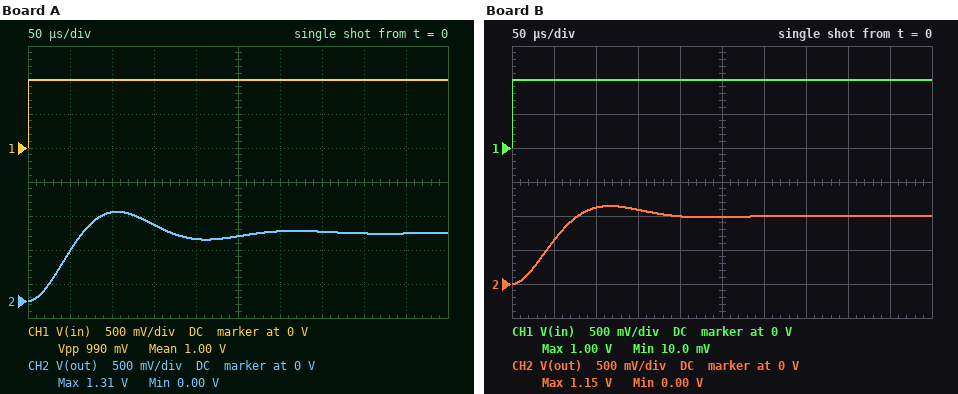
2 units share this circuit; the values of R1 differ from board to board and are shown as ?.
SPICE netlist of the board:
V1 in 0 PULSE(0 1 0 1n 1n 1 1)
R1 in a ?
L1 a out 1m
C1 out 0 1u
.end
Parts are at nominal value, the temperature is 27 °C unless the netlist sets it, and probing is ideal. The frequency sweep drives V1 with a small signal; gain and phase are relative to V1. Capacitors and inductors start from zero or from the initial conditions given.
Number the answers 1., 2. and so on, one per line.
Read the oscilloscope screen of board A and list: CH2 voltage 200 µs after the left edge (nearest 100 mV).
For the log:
1. 900 mV
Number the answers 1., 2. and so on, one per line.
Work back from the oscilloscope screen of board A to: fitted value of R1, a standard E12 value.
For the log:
1. 22 Ω
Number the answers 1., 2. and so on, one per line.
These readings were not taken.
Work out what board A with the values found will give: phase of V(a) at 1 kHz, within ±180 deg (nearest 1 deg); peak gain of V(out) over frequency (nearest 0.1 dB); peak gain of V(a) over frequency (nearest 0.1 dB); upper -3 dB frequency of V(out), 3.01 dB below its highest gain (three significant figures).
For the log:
1. -8 deg
2. 3.7 dB
3. 0 dB
4. 5.98 kHz
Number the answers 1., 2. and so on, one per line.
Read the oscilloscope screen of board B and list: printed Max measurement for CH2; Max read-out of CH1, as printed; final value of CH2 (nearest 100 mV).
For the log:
1. 1.15 V
2. 1.00 V
3. 1.0 V
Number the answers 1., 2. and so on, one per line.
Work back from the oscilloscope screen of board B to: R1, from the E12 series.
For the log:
1. 33 Ω
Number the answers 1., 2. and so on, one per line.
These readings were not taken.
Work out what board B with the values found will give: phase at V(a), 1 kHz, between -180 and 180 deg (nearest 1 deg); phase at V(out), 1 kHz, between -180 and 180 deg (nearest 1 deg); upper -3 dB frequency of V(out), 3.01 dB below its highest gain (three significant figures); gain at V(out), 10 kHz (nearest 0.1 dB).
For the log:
1. -12 deg
2. -12 deg
3. 5.84 kHz
4. -11.1 dB
